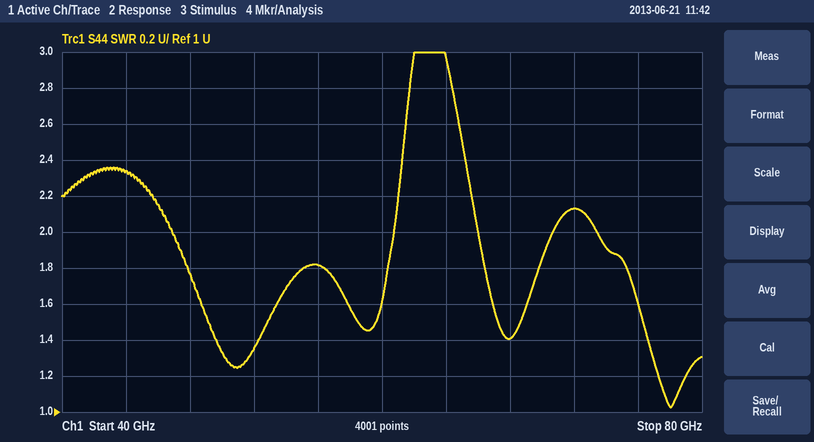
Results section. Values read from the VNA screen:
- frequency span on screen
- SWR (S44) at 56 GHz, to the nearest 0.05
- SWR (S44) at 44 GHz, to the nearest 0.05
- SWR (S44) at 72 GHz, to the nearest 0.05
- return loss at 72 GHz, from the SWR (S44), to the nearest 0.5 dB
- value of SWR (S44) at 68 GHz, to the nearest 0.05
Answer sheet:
40 GHz
1.80
2.35
2.15
9.0 dB
1.40
